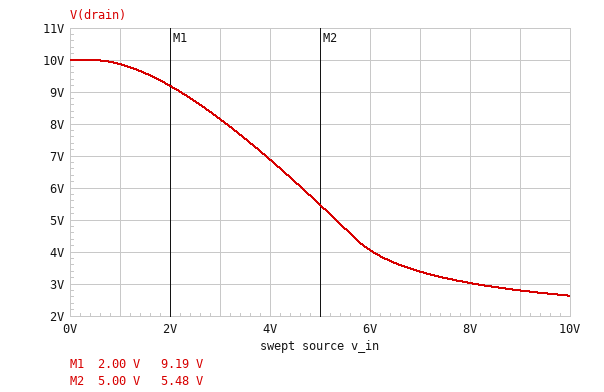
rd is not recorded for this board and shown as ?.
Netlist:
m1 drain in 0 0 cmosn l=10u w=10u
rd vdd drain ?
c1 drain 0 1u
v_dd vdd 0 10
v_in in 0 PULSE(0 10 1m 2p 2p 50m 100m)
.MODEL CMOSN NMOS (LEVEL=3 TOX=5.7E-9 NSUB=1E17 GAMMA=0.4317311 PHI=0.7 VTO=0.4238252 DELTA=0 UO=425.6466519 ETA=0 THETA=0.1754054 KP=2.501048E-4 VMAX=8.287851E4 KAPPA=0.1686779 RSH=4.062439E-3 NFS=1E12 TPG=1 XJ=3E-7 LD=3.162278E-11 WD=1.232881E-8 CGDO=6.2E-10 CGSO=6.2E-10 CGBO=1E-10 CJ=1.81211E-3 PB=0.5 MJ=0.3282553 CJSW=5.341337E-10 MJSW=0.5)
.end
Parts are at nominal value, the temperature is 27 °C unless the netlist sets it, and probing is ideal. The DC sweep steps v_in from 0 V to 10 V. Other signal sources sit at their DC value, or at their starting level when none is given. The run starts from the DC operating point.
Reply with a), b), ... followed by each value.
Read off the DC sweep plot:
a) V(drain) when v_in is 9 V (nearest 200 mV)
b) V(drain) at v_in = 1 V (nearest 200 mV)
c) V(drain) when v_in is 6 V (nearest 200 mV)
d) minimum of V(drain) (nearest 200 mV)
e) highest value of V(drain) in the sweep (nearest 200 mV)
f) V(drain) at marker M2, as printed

a) 2.8 V
b) 9.8 V
c) 4.0 V
d) 2.6 V
e) 10.0 V
f) 5.48 V
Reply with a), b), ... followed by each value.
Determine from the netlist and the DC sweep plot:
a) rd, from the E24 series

a) 3.9 kΩ
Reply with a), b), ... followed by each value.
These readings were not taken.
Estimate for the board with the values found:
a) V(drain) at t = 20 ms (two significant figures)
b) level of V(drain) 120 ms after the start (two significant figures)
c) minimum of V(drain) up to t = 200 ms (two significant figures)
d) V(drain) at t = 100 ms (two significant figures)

a) 2.6 V
b) 2.6 V
c) 2.6 V
d) 10 V
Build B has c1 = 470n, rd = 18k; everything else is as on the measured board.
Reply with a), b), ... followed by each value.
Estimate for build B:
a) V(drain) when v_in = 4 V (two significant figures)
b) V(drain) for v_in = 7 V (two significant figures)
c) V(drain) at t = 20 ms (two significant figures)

a) 1.1 V
b) 730 mV
c) 610 mV
